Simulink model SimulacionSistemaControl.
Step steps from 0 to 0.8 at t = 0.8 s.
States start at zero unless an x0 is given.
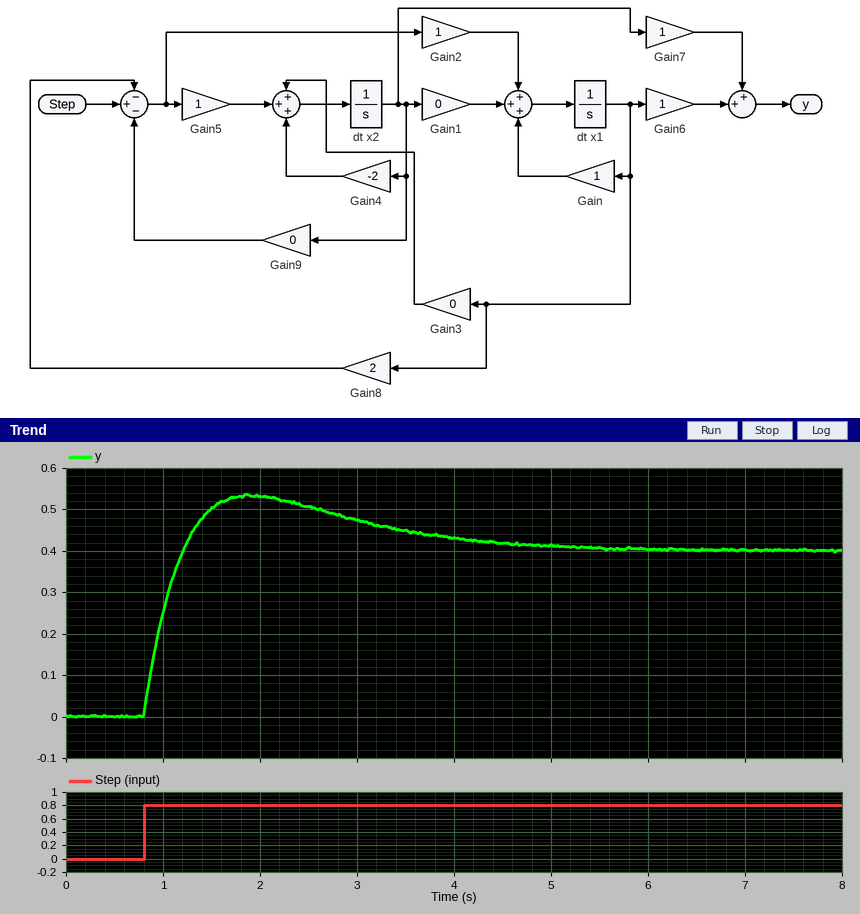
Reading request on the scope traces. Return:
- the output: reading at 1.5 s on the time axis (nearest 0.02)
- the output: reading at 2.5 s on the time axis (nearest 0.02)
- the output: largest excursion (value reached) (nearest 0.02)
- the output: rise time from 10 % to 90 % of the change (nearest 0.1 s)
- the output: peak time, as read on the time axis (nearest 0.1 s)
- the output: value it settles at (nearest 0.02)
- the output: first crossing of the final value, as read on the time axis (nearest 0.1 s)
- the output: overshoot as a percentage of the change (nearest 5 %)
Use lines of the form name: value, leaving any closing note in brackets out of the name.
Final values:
the output: reading at 1.5 s on the time axis: 0.50
the output: reading at 2.5 s on the time axis: 0.50
the output: largest excursion (value reached): 0.54
the output: rise time from 10 % to 90 % of the change: 0.3 s
the output: peak time, as read on the time axis: 1.9 s
the output: value it settles at: 0.40
the output: first crossing of the final value, as read on the time axis: 1.2 s
the output: overshoot as a percentage of the change: 35 %
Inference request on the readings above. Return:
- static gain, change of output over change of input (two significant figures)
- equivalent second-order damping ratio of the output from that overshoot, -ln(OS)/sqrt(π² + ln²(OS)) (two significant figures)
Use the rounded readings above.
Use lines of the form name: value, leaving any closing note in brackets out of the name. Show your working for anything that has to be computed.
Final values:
static gain, change of output over change of input: (0.4 - 0) / (0.8 - 0) = 0.50
equivalent second-order damping ratio of the output from that overshoot, -ln(OS)/sqrt(π² + ln²(OS)): ln(0.35) = -1.050; 1.050 / sqrt(9.870 + 1.102) = 0.32
